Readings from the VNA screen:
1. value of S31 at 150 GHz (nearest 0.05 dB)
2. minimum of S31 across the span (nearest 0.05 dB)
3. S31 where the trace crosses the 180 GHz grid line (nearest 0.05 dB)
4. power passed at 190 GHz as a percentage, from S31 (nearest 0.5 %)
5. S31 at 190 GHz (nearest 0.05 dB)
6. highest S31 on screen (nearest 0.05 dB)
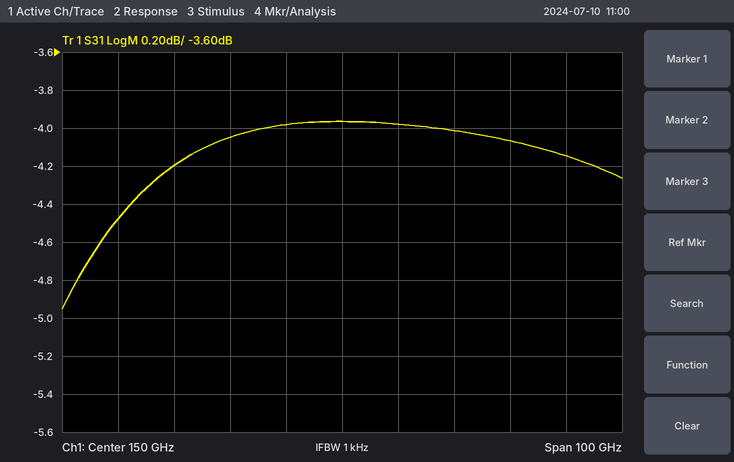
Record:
-3.95 dB
-4.95 dB
-4.05 dB
38.5 %
-4.15 dB
-3.95 dB
